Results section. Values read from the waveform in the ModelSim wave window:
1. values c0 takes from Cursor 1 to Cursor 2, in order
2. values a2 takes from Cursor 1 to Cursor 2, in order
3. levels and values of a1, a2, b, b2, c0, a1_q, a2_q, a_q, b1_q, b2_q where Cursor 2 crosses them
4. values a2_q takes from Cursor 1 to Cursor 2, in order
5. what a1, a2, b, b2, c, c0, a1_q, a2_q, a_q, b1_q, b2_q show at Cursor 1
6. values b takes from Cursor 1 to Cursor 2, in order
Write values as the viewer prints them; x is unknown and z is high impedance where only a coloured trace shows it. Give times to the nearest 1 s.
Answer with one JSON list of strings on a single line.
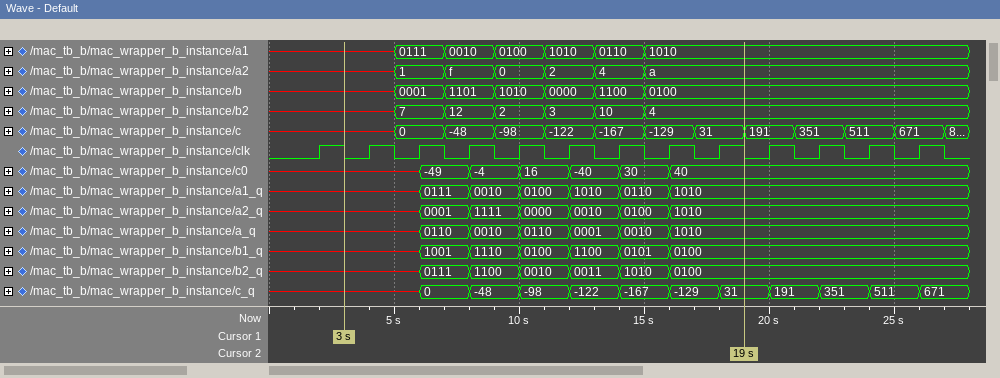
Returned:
["x, -49, -4, 16, -40, 30, 40", "x, 1, f, 0, 2, 4, a", "a1=1010, a2=a, b=0100, b2=4, c0=40, a1_q=1010, a2_q=1010, a_q=1010, b1_q=0100, b2_q=0100", "x, 0001, 1111, 0000, 0010, 0100, 1010", "a1=x, a2=x, b=x, b2=x, c=x, c0=x, a1_q=x, a2_q=x, a_q=x, b1_q=x, b2_q=x", "x, 0001, 1101, 1010, 0000, 1100, 0100"]
